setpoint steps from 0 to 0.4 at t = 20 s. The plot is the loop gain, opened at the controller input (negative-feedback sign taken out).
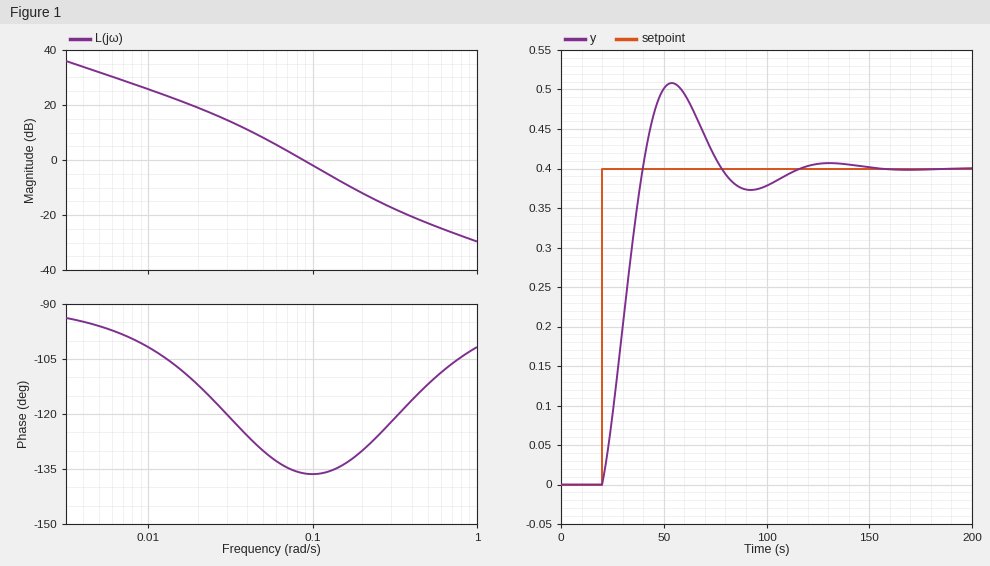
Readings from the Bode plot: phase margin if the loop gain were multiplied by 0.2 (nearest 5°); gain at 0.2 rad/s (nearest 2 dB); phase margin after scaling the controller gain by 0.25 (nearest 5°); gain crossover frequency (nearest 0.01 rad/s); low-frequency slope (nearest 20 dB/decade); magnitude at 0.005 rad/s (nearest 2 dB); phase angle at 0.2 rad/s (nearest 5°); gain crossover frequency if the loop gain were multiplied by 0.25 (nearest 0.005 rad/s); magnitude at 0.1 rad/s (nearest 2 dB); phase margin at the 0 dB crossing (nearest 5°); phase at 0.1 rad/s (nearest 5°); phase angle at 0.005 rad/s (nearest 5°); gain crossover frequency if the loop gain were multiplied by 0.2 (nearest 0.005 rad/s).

60°
-12 dB
55°
0.09 rad/s
-20 dB/decade
32 dB
-130°
0.035 rad/s
-2 dB
45°
-135°
-95°
0.030 rad/s
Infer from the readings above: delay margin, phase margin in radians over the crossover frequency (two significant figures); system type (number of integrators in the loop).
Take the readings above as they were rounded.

8.7 s
1
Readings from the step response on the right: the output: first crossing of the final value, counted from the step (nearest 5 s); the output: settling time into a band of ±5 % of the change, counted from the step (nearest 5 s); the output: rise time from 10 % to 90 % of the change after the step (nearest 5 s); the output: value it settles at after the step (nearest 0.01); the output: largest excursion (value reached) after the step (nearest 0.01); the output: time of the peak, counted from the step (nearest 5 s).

20 s
80 s
15 s
0.40
0.51
35 s
